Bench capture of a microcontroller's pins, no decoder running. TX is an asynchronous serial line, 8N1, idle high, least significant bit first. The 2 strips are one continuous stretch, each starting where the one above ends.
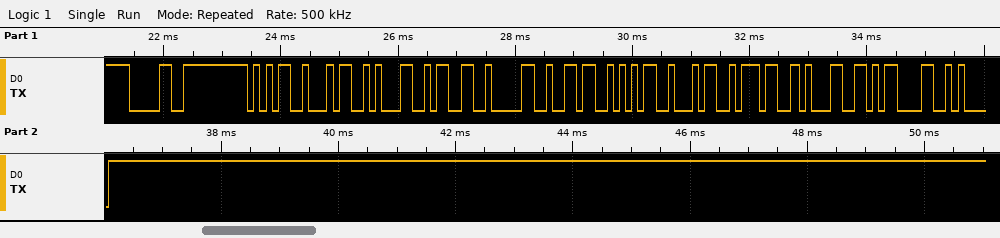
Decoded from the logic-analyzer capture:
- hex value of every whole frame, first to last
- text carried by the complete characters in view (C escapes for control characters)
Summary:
30 35 34 31 33 30 36 35 34 37 31 0D 0A
"05413065471\r\n"
